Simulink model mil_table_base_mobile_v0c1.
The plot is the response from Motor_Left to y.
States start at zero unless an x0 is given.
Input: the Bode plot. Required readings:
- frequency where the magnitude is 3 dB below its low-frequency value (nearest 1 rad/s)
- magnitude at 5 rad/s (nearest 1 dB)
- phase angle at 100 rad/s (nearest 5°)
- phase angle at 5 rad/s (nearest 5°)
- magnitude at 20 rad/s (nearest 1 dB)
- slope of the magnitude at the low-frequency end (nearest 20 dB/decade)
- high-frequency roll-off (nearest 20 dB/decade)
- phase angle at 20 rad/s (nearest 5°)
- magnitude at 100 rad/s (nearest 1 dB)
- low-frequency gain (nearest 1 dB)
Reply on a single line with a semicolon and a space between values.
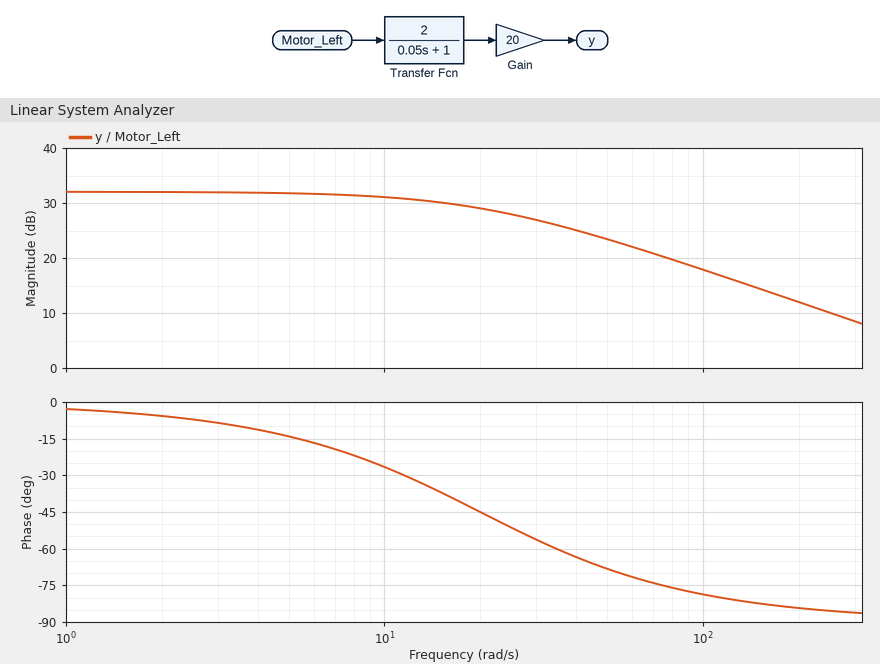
20 rad/s; 32 dB; -80°; -15°; 29 dB; 0 dB/decade; -20 dB/decade; -45°; 18 dB; 32 dB
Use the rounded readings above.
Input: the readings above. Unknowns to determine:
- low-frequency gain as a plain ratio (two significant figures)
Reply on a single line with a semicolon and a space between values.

40
